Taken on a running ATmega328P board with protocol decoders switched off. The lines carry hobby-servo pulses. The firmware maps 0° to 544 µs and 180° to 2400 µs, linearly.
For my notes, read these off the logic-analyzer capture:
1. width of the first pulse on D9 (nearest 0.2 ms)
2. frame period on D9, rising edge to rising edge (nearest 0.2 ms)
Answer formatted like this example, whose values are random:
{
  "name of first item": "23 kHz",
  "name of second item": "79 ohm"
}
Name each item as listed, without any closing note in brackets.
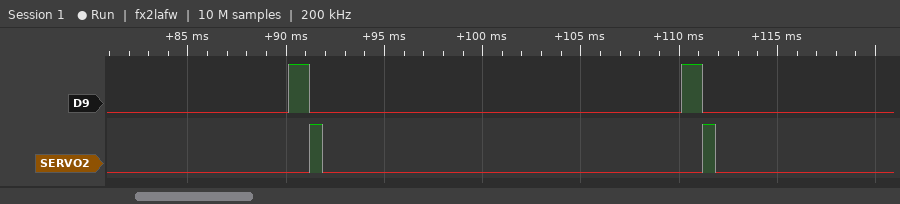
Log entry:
{
  "width of the first pulse on D9": "1.0 ms",
  "frame period on D9, rising edge to rising edge": "20.0 ms"
}
